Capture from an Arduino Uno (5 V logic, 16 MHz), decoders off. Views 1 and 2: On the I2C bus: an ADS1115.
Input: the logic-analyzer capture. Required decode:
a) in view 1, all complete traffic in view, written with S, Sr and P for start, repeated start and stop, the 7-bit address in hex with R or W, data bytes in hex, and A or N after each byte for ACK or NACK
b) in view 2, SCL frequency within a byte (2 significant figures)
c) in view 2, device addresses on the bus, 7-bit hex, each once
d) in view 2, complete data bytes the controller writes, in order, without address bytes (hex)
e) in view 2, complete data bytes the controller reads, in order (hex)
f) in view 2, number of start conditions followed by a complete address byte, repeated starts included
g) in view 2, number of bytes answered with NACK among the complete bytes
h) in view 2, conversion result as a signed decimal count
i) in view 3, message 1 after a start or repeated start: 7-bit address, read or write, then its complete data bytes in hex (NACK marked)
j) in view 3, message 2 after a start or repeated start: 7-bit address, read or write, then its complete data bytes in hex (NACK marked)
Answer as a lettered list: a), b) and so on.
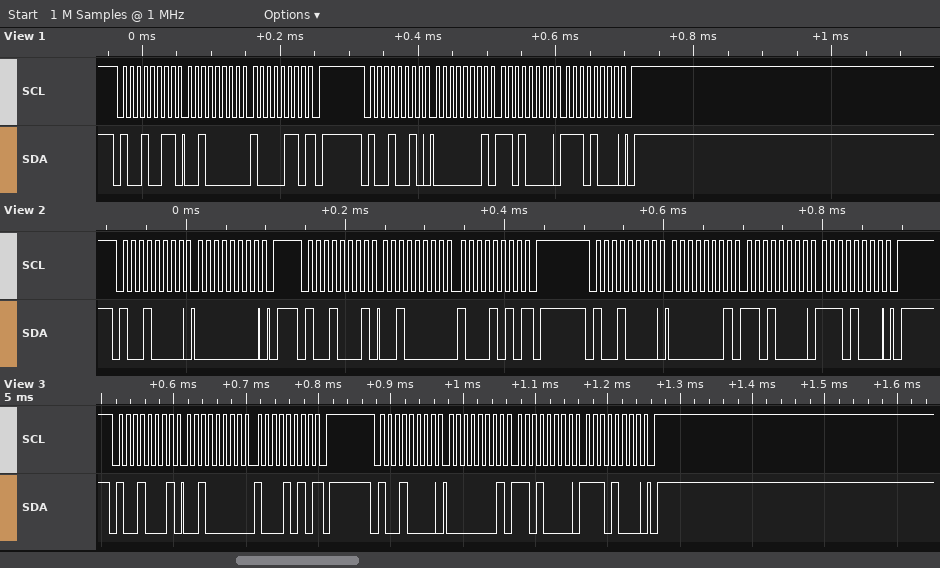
a) S 49R A 20 A 86 N P S 49W A 01 A D0 A E8 A P
b) 100 kHz
c) 0x48
d) 00 01 D0 E8
e) 20 8A
f) 3
g) 1
h) 8330
i) 0x48 read: 20 8A NACK
j) 0x48 write: 01 D0 E8
